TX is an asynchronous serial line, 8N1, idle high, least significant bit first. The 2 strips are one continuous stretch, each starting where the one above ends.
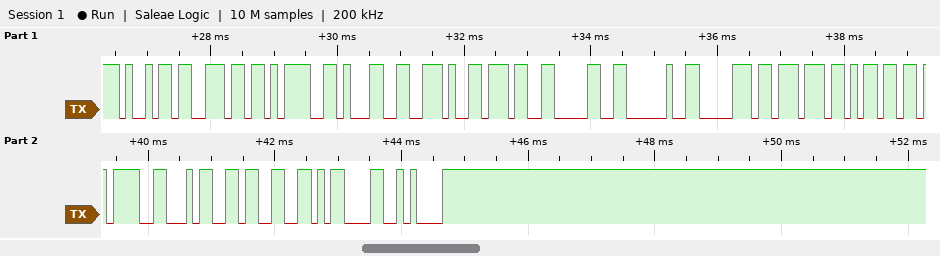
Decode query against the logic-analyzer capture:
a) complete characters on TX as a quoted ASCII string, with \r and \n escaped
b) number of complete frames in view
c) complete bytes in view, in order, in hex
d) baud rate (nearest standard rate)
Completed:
"in=1.70 pwm=43\r\n"
16
69 6E 3D 31 2E 37 30 20 70 77 6D 3D 34 33 0D 0A
9600 baud
